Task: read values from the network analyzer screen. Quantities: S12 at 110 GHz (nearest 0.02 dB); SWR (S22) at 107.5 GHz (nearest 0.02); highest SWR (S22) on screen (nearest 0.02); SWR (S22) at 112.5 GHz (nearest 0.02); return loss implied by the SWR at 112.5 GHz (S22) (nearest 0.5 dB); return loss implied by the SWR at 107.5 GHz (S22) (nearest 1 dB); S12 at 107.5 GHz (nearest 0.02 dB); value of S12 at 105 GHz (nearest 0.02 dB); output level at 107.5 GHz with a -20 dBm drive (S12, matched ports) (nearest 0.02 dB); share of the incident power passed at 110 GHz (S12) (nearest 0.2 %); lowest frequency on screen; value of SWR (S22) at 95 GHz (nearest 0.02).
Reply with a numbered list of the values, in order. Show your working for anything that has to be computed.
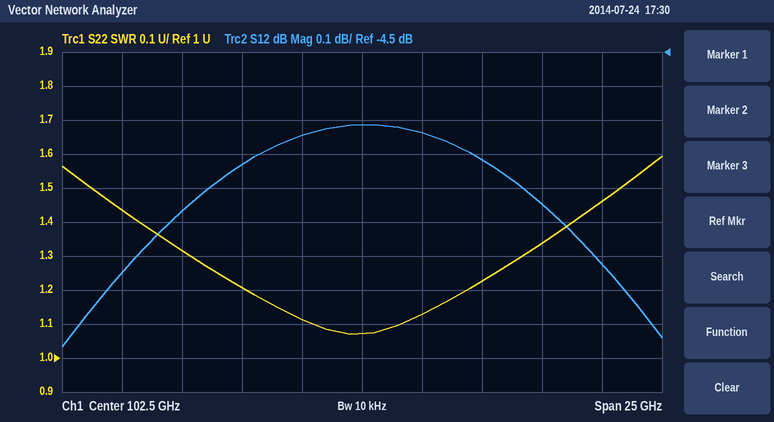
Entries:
1. -4.94 dB
2. 1.22
3. 1.60
4. 1.46
5. −20 log10((1.46 − 1)/(1.46 + 1)) ≈ 14.6 dB, so 14.5 dB to the nearest 0.5 dB
6. −20 log10((1.22 − 1)/(1.22 + 1)) ≈ 20 dB
7. -4.82 dB
8. -4.74 dB
9. -20 dBm + (-4.82 dB) = -24.82 dBm
10. 10^(-4.94/10) ≈ 32.1 %, so 32.0 % to the nearest 0.2 %
11. 90 GHz
12. 1.32
